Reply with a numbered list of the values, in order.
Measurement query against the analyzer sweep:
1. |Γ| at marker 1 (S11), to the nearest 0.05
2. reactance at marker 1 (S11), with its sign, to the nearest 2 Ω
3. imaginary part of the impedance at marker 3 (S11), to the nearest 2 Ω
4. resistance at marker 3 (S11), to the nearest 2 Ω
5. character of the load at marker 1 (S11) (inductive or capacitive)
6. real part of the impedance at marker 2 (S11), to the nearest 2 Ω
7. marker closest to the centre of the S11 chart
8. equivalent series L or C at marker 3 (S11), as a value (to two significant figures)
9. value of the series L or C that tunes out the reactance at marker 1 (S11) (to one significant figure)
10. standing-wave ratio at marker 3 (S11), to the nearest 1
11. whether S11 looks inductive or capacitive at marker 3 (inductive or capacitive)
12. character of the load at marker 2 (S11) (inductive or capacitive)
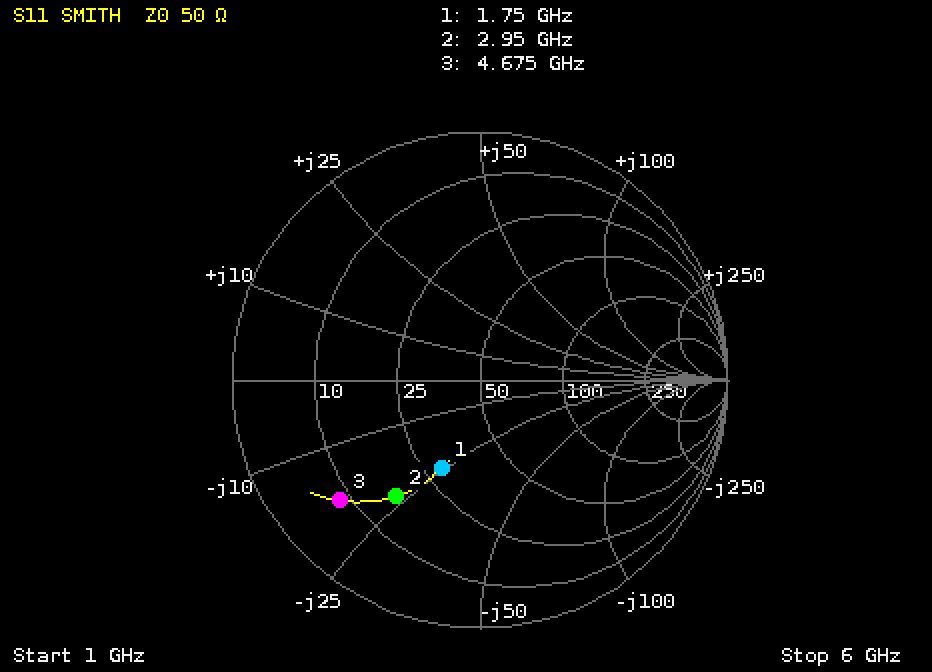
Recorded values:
1. 0.40
2. -24 Ω
3. -18 Ω
4. 8 Ω
5. capacitive
6. 16 Ω
7. marker 1
8. 1.9 pF
9. 2 nH
10. 7
11. capacitive
12. capacitive
